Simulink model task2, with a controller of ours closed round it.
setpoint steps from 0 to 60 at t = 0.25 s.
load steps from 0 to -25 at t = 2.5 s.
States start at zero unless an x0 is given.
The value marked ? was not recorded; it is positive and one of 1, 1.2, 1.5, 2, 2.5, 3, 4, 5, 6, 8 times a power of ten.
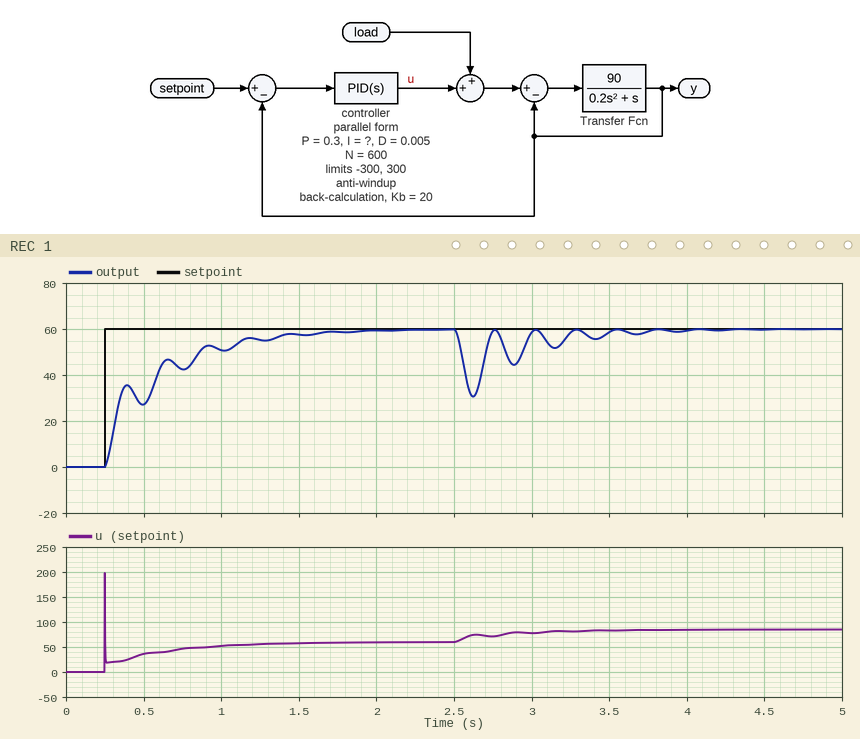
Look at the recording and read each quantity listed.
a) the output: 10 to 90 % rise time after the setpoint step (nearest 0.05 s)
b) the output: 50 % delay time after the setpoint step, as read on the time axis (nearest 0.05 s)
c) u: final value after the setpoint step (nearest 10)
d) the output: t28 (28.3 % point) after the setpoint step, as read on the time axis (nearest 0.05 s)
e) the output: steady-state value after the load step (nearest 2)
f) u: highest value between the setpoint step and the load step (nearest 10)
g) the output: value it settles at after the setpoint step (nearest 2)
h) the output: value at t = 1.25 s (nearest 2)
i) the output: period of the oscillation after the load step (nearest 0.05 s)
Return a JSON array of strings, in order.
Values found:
["0.85 s", "0.35 s", "60", "0.30 s", "60", "200", "60", "56", "0.25 s"]
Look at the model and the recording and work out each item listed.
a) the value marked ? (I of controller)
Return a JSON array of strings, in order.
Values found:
["3"]
